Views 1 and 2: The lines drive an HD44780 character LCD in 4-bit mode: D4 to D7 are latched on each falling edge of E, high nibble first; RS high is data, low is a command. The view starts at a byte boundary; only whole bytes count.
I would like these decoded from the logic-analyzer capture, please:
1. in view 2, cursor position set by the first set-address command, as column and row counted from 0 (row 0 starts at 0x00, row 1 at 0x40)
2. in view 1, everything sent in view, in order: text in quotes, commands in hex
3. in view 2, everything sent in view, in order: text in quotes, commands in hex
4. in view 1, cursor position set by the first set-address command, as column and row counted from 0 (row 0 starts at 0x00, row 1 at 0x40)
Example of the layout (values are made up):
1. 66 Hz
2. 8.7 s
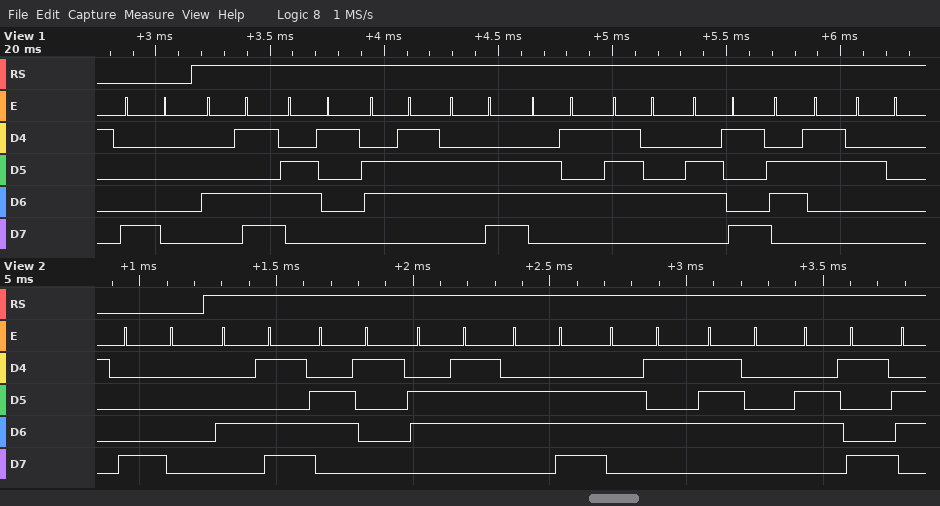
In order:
1. column 0, row 0
2. 0x80 "Magnetic "
3. 0x80 "Magneti"
4. column 0, row 0
